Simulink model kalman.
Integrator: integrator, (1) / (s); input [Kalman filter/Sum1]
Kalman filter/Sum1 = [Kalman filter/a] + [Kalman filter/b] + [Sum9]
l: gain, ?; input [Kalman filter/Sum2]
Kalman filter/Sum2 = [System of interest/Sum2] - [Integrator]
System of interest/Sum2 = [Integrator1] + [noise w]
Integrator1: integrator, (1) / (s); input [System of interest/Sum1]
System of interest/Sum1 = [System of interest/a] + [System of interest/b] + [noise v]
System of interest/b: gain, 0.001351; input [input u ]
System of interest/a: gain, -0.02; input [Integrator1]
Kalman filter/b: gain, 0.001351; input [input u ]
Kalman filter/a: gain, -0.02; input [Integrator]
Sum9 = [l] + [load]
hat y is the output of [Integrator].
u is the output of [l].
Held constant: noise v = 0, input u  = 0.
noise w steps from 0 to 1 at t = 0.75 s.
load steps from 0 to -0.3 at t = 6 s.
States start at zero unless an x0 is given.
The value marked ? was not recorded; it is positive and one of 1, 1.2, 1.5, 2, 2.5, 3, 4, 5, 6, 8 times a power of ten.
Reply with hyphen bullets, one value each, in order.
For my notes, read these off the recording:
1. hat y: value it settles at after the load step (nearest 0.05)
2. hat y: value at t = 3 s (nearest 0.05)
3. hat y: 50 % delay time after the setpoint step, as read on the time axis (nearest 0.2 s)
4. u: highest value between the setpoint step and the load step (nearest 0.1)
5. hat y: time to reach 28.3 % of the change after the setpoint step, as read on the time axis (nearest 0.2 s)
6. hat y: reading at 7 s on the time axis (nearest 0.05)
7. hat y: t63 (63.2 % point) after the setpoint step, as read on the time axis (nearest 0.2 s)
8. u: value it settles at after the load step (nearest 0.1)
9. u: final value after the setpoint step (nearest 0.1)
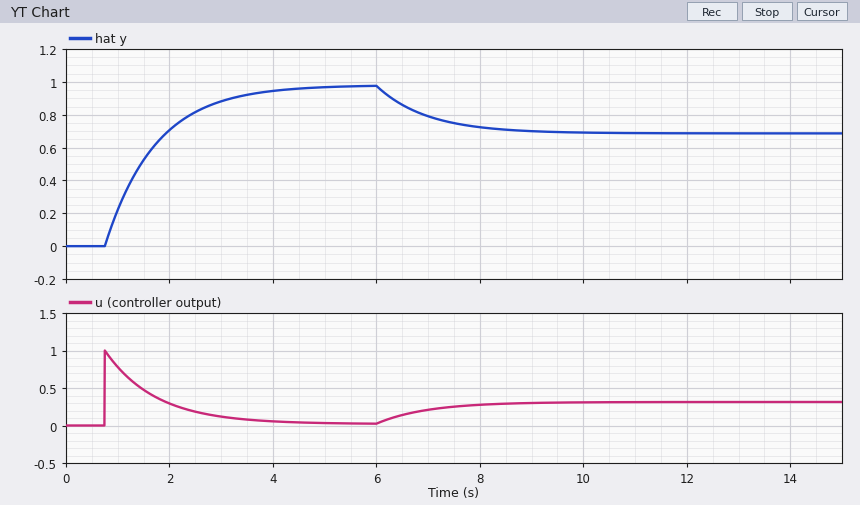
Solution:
- 0.70
- 0.90
- 1.4 s
- 1.0
- 1.0 s
- 0.80
- 1.8 s
- 0.3
- 0.0
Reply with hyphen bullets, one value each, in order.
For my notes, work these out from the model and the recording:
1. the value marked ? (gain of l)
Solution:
- 1
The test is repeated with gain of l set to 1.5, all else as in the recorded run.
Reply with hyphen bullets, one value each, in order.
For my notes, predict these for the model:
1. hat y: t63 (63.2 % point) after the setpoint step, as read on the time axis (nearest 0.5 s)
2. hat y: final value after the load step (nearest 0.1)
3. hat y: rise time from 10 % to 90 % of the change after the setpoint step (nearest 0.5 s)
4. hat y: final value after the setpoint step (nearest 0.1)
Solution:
- 1.5 s
- 0.8
- 1.5 s
- 1.0
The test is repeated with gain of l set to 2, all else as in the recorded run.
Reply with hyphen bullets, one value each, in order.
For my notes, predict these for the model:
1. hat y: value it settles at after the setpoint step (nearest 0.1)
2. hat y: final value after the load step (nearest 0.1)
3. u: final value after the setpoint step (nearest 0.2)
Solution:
- 1.0
- 0.8
- 0.0
